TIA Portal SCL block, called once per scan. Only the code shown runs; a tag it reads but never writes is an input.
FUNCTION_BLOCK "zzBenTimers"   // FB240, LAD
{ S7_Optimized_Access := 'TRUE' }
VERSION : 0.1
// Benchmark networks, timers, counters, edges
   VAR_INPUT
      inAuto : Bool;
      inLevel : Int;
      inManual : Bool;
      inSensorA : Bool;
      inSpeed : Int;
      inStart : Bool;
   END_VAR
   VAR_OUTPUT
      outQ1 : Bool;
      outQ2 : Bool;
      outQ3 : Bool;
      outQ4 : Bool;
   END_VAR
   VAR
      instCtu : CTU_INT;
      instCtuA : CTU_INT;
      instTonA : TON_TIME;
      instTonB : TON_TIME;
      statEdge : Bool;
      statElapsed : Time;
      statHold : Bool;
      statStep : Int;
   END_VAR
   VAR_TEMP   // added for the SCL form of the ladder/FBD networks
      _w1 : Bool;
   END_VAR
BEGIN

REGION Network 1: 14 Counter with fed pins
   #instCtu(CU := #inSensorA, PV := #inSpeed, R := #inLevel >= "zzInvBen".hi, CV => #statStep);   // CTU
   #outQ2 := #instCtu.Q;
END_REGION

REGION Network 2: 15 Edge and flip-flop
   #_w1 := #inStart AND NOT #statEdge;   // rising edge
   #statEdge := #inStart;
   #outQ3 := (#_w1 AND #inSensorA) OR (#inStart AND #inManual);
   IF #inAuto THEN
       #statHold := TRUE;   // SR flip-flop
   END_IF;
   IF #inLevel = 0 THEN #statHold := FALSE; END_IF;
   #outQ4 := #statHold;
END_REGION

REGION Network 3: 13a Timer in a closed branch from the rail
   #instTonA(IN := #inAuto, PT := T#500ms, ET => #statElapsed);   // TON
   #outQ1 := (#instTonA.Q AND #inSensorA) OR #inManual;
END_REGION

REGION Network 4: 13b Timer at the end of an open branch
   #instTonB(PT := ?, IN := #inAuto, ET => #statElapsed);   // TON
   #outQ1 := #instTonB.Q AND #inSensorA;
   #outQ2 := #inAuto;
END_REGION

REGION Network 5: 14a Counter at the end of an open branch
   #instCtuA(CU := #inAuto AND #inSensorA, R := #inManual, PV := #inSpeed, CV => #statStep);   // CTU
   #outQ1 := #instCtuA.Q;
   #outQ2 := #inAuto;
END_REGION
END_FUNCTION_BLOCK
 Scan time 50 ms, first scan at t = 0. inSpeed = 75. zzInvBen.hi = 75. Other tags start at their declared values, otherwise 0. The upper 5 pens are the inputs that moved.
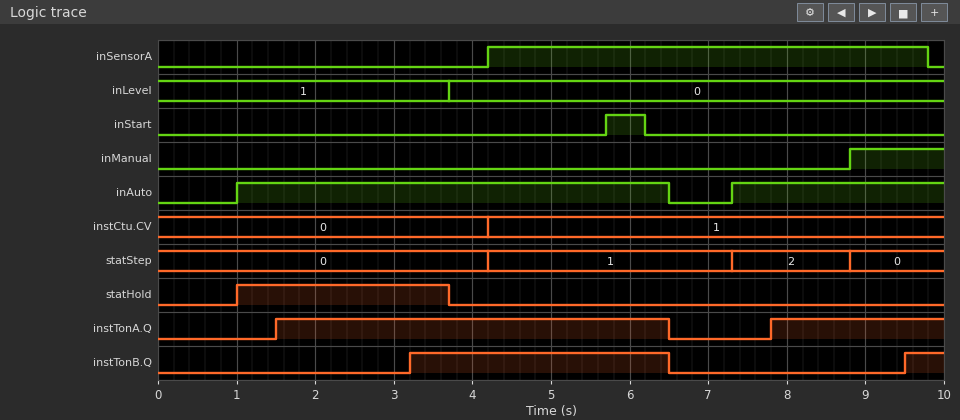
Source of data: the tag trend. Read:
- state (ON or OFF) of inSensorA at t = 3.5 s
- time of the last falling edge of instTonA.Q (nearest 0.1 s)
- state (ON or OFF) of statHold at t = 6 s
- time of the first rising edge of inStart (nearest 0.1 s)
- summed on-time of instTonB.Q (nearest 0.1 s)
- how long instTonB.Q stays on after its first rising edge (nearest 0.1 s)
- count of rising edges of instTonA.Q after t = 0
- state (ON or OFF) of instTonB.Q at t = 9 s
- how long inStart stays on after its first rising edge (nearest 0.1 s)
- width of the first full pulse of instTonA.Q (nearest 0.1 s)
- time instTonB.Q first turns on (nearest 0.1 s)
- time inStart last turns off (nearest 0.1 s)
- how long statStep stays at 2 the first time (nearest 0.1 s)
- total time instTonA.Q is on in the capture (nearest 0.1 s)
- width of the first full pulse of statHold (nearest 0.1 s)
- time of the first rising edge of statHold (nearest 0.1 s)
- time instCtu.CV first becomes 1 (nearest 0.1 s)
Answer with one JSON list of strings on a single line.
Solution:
["OFF", "6.5 s", "OFF", "5.7 s", "3.8 s", "3.3 s", "2", "OFF", "0.5 s", "5.0 s", "3.2 s", "6.2 s", "1.5 s", "7.2 s", "2.7 s", "1.0 s", "4.2 s"]
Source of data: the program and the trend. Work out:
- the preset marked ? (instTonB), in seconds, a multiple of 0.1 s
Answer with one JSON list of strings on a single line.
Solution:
["2.2 s"]
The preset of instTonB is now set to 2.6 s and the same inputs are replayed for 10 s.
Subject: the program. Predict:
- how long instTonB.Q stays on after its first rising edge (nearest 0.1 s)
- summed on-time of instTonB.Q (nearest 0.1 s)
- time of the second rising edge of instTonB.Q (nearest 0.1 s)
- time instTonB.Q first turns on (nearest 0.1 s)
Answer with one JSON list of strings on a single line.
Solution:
["2.9 s", "3.0 s", "9.9 s", "3.6 s"]
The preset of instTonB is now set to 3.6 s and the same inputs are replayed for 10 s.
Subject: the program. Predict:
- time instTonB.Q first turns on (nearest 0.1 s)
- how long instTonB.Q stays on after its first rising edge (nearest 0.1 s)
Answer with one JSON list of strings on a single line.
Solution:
["4.6 s", "1.9 s"]
